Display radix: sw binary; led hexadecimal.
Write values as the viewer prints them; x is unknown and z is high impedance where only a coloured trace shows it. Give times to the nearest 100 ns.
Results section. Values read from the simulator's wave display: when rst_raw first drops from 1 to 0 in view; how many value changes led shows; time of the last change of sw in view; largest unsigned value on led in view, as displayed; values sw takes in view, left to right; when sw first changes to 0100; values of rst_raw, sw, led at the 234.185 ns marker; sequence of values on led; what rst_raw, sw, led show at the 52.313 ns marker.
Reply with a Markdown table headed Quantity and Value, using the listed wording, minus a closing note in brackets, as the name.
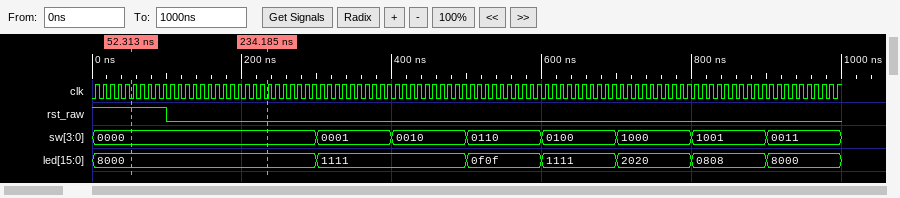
| Quantity | Value |
|---|---|
| when rst_raw first drops from 1 to 0 in view | 100 ns |
| how many value changes led shows | 6 |
| time of the last change of sw in view | 900 ns |
| largest unsigned value on led in view, as displayed | 8000 |
| values sw takes in view, left to right | 0000, 0001, 0010, 0110, 0100, 1000, 1001, 0011 |
| when sw first changes to 0100 | 600 ns |
| values of rst_raw, sw, led at the 234.185 ns marker | rst_raw=0, sw=0000, led=8000 |
| sequence of values on led | 8000, 1111, 0f0f, 1111, 2020, 0808, 8000 |
| what rst_raw, sw, led show at the 52.313 ns marker | rst_raw=1, sw=0000, led=8000 |
